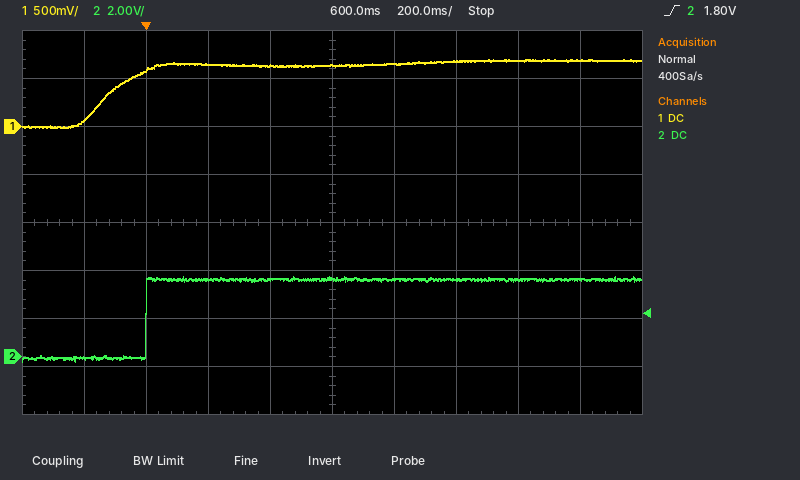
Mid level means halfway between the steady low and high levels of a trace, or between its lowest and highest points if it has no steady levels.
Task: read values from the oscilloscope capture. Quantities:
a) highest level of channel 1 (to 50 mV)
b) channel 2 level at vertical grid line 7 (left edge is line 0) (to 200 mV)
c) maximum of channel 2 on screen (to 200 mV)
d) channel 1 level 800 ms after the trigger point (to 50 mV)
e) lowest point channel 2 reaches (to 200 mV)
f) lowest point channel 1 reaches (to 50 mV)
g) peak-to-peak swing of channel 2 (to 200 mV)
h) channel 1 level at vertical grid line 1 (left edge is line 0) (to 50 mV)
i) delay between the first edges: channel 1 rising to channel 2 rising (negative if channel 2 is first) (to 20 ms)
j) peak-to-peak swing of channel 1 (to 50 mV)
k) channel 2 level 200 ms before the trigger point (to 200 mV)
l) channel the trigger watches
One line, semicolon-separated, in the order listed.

700 mV; 3.2 V; 3.4 V; 650 mV; -200 mV; 0 mV; 3.6 V; 50 mV; +120 ms; 700 mV; 0.0 V; channel 2
